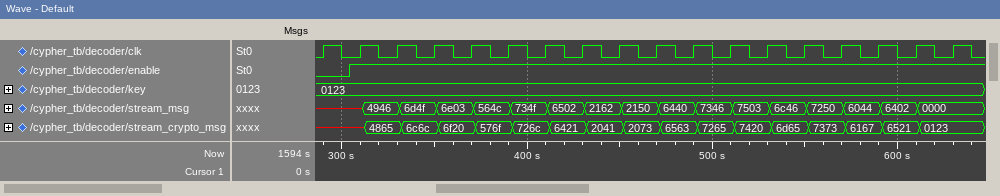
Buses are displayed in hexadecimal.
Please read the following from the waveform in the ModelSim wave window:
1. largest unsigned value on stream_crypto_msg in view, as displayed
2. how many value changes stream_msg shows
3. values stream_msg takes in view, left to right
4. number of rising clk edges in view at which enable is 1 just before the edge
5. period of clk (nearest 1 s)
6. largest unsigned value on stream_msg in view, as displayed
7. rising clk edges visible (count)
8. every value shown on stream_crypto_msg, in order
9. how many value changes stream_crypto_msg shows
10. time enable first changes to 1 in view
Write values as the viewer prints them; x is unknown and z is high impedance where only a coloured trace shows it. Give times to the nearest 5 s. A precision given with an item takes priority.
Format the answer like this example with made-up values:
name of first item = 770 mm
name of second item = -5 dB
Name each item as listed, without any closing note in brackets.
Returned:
largest unsigned value on stream_crypto_msg in view, as displayed = 7420
how many value changes stream_msg shows = 16
values stream_msg takes in view, left to right = x, 4946, 6d4f, 6e03, 564c, 734f, 6502, 2162, 2150, 6440, 7346, 7503, 6c46, 7250, 6044, 6402, 0000
number of rising clk edges in view at which enable is 1 just before the edge = 17
period of clk = 20 s
largest unsigned value on stream_msg in view, as displayed = 7503
rising clk edges visible = 18
every value shown on stream_crypto_msg, in order = x, 4865, 6c6c, 6f20, 576f, 726c, 6421, 2041, 2073, 6563, 7265, 7420, 6d65, 7373, 6167, 6521, 0123
how many value changes stream_crypto_msg shows = 16
time enable first changes to 1 in view = 305 s
